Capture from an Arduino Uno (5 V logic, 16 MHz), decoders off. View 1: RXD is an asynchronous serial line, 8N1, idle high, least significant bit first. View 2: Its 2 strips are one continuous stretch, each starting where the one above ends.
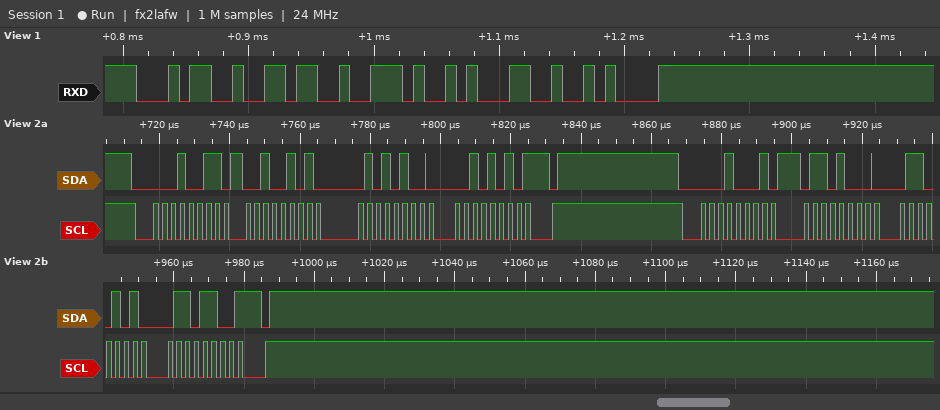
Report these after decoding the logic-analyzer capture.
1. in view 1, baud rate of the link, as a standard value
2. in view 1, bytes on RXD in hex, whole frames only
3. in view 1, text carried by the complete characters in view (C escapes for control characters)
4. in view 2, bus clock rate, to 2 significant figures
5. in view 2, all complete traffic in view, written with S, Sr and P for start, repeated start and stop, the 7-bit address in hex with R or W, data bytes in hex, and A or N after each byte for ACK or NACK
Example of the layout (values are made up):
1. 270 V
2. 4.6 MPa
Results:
1. 115200 baud
2. 34 36 2E 31 0A
3. "46.1\n"
4. 400 kHz
5. S 09R A 25 A 54 A 2A N P S 08R A 68 A 65 A 6C N P
